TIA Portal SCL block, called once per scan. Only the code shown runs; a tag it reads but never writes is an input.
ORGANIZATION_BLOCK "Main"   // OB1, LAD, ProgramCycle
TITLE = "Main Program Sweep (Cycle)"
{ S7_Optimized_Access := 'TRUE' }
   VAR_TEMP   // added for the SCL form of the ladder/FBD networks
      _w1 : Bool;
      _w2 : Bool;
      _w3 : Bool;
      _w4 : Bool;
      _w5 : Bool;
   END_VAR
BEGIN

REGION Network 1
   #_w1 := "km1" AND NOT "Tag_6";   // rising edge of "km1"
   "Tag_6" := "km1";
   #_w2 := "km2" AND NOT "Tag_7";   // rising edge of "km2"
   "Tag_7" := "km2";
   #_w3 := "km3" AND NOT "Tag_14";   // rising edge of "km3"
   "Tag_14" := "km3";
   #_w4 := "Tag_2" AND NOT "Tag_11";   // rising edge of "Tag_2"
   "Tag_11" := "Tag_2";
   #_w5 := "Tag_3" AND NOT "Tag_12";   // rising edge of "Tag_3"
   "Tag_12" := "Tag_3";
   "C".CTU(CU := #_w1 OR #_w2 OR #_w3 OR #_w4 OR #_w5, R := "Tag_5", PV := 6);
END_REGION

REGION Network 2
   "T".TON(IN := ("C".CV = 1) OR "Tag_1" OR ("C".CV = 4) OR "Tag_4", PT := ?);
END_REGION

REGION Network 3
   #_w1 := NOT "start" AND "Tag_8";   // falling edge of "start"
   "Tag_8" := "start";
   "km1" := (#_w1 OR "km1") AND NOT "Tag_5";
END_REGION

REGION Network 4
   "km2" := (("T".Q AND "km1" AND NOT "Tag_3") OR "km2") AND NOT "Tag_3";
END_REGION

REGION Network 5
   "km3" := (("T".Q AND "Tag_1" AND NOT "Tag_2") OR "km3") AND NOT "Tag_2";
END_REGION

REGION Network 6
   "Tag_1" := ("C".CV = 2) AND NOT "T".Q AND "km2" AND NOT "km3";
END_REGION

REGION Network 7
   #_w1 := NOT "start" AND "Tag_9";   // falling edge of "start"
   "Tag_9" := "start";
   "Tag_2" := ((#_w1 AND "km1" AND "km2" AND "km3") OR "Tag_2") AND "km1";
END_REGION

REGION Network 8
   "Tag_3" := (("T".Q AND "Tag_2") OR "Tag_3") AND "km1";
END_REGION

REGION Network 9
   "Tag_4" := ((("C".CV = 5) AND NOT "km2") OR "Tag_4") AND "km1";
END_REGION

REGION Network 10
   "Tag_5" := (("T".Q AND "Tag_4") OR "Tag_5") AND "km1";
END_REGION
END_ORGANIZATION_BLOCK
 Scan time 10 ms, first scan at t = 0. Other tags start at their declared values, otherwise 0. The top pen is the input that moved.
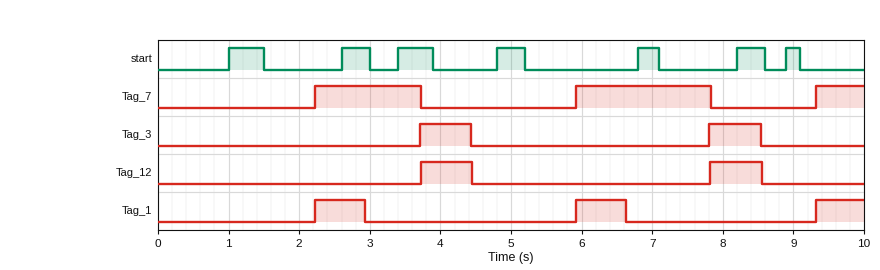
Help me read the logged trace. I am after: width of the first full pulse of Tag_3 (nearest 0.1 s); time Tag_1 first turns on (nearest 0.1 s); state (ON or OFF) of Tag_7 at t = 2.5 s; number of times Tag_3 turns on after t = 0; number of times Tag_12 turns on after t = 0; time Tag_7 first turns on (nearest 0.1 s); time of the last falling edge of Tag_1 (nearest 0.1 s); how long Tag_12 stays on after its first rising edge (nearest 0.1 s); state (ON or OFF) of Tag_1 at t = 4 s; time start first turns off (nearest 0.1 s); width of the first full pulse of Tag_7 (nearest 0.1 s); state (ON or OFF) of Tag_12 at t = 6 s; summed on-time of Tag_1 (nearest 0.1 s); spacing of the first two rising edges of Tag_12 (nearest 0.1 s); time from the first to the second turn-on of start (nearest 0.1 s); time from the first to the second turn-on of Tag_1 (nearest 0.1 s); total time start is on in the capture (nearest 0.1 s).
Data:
0.7 s
2.2 s
ON
2
2
2.2 s
6.6 s
0.7 s
OFF
1.5 s
1.5 s
OFF
2.1 s
4.1 s
1.6 s
3.7 s
2.7 s
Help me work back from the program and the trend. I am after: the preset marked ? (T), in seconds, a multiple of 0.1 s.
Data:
0.7 s
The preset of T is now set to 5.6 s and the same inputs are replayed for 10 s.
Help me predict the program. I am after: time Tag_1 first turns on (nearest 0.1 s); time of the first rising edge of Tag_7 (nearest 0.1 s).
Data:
7.1 s
7.1 s
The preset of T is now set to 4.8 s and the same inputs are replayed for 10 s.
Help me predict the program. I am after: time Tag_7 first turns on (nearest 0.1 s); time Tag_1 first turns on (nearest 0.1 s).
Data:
6.3 s
6.3 s
